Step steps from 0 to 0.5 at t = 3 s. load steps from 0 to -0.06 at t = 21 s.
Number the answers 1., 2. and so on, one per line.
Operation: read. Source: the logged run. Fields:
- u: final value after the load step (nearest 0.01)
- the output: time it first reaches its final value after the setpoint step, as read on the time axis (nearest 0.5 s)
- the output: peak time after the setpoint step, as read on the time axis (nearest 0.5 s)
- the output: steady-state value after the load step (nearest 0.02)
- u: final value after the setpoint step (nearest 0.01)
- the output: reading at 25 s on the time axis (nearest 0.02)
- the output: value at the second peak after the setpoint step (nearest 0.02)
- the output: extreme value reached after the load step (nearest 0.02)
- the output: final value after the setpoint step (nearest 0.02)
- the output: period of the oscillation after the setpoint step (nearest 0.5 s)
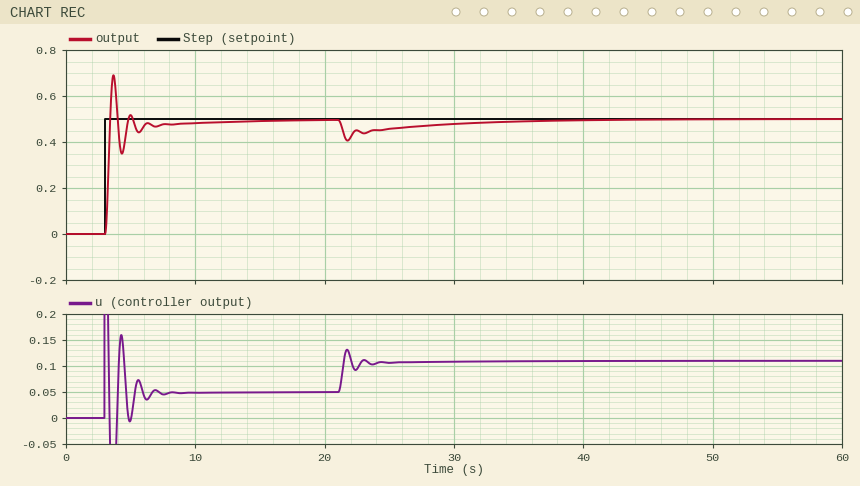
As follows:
1. 0.11
2. 3.5 s
3. 3.5 s
4. 0.50
5. 0.05
6. 0.46
7. 0.52
8. 0.40
9. 0.50
10. 1.5 s
